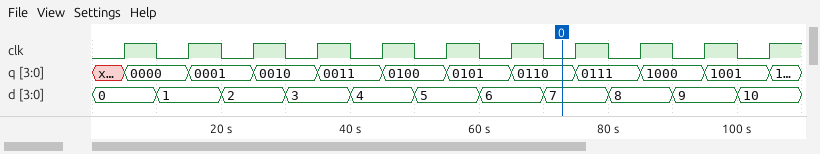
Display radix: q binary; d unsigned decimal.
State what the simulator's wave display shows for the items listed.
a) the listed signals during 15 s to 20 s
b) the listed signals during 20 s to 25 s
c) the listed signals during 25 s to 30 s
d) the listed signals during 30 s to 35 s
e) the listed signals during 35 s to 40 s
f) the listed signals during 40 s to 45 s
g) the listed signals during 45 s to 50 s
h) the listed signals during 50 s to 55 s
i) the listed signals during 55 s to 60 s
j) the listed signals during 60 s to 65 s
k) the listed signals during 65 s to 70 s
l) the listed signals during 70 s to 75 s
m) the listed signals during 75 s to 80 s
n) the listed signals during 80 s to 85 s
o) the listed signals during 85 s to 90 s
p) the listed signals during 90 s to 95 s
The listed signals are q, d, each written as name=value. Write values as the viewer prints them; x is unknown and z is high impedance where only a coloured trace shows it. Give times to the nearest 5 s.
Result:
q=0001, d=1
q=0001, d=2
q=0010, d=2
q=0010, d=3
q=0011, d=3
q=0011, d=4
q=0100, d=4
q=0100, d=5
q=0101, d=5
q=0101, d=6
q=0110, d=6
q=0110, d=7
q=0111, d=7
q=0111, d=8
q=1000, d=8
q=1000, d=9
